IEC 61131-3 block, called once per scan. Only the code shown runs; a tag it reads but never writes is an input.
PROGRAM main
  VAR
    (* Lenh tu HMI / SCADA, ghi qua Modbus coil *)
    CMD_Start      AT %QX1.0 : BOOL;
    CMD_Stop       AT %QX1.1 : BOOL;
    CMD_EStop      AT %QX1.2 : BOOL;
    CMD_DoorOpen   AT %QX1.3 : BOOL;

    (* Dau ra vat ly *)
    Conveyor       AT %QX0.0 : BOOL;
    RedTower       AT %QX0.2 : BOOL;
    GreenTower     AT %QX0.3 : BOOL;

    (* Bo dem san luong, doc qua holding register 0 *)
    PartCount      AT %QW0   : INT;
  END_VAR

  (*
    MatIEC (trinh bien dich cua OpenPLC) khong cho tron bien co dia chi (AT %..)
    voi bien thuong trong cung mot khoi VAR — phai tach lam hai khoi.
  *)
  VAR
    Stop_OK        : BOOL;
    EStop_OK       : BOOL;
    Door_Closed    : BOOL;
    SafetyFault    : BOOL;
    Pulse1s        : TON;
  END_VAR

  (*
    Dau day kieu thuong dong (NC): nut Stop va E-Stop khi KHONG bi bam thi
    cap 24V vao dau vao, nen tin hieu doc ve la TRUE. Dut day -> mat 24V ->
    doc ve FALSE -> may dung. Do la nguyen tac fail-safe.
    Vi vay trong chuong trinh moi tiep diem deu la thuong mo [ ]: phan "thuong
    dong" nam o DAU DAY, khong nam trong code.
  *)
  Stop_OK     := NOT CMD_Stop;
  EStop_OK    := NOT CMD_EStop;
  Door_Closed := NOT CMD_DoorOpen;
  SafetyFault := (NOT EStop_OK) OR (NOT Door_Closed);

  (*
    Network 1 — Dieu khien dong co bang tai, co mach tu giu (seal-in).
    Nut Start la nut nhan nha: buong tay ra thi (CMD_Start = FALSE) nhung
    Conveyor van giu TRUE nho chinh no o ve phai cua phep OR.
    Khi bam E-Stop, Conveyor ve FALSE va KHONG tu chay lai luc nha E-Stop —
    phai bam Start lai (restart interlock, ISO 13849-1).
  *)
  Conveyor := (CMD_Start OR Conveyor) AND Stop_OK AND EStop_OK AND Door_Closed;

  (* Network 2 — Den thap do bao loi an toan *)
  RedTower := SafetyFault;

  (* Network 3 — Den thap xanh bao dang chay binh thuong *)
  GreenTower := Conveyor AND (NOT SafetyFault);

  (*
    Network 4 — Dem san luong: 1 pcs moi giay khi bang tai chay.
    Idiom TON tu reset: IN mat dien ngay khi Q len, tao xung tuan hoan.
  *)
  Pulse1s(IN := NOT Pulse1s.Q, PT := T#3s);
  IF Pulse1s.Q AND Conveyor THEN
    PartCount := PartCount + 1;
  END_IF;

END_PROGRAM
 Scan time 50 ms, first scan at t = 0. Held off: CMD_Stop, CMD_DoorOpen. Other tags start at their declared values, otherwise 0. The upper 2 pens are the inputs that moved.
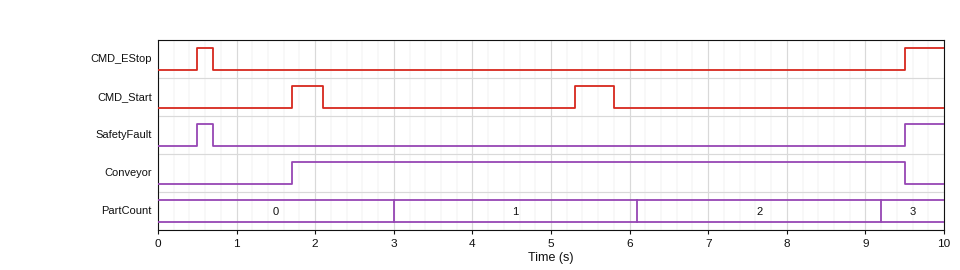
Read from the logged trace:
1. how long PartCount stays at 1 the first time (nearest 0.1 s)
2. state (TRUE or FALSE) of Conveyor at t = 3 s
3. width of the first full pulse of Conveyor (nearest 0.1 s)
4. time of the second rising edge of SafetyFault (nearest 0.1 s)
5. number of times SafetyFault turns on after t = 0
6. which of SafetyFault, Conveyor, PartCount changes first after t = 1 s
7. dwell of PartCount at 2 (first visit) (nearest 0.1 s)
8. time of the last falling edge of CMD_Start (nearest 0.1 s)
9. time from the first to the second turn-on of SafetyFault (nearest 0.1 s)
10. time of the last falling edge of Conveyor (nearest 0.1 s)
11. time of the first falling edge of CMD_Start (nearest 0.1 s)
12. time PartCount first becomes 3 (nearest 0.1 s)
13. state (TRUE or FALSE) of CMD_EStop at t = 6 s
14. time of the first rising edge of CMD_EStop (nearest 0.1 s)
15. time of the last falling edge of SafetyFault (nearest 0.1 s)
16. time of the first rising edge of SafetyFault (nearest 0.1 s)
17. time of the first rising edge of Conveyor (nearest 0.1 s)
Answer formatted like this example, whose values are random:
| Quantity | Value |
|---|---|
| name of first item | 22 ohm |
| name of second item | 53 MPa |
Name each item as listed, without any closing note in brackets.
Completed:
| Quantity | Value |
|---|---|
| how long PartCount stays at 1 the first time | 3.1 s |
| state (TRUE or FALSE) of Conveyor at t = 3 s | TRUE |
| width of the first full pulse of Conveyor | 7.8 s |
| time of the second rising edge of SafetyFault | 9.5 s |
| number of times SafetyFault turns on after t = 0 | 2 |
| which of SafetyFault, Conveyor, PartCount changes first after t = 1 s | Conveyor |
| dwell of PartCount at 2 (first visit) | 3.1 s |
| time of the last falling edge of CMD_Start | 5.8 s |
| time from the first to the second turn-on of SafetyFault | 9.0 s |
| time of the last falling edge of Conveyor | 9.5 s |
| time of the first falling edge of CMD_Start | 2.1 s |
| time PartCount first becomes 3 | 9.2 s |
| state (TRUE or FALSE) of CMD_EStop at t = 6 s | FALSE |
| time of the first rising edge of CMD_EStop | 0.5 s |
| time of the last falling edge of SafetyFault | 0.7 s |
| time of the first rising edge of SafetyFault | 0.5 s |
| time of the first rising edge of Conveyor | 1.7 s |
